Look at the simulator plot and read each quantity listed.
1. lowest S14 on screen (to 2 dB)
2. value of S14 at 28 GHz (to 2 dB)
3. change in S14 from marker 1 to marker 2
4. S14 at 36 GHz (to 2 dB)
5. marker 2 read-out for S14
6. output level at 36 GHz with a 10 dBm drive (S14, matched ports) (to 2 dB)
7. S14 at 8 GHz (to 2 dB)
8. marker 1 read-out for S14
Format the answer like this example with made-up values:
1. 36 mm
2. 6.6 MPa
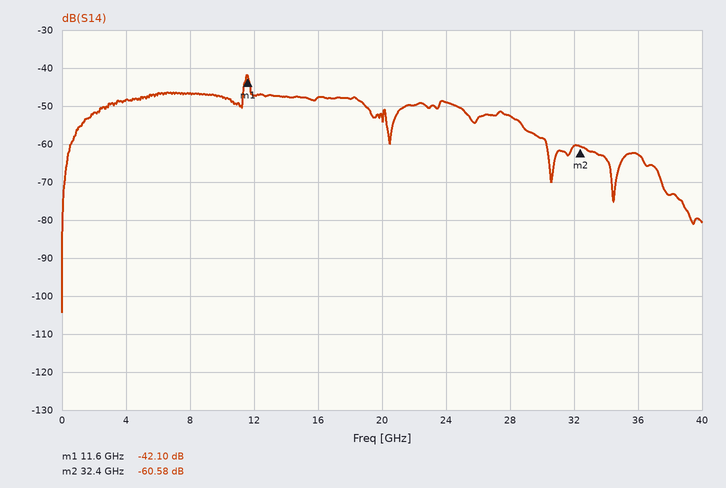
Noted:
1. -104 dB
2. -52 dB
3. -18.48 dB
4. -62 dB
5. -60.58 dB
6. -52 dBm
7. -46 dB
8. -42.10 dB
